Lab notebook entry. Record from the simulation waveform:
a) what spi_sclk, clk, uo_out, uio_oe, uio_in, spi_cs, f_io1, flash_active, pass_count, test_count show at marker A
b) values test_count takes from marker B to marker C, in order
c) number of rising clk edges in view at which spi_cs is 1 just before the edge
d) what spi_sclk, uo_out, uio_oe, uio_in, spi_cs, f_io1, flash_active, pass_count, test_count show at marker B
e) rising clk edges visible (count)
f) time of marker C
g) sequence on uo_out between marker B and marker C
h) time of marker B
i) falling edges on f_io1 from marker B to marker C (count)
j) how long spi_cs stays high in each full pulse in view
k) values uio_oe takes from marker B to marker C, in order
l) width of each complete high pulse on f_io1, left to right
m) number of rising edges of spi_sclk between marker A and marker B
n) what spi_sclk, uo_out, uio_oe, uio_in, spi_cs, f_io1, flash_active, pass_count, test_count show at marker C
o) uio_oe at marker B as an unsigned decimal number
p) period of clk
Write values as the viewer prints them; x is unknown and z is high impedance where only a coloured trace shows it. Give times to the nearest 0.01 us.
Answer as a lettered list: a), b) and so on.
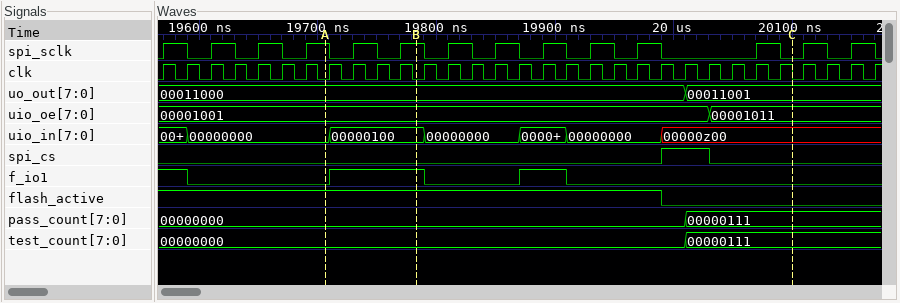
a) spi_sclk=1, clk=0, uo_out=00011000, uio_oe=00001001, uio_in=00000000, spi_cs=0, f_io1=0, flash_active=1, pass_count=00000000, test_count=00000000
b) 00000000, 00000111
c) 2
d) spi_sclk=1, uo_out=00011000, uio_oe=00001001, uio_in=00000100, spi_cs=0, f_io1=1, flash_active=1, pass_count=00000000, test_count=00000000
e) 31
f) 20.1 us
g) 00011000, 00011001
h) 19.78 us
i) 2
j) 0.04 us
k) 00001001, 00001011
l) 0.08 us, 0.04 us
m) 2
n) spi_sclk=0, uo_out=00011001, uio_oe=00001011, uio_in=00000z00, spi_cs=0, f_io1=0, flash_active=0, pass_count=00000111, test_count=00000111
o) 9
p) 0.02 us
